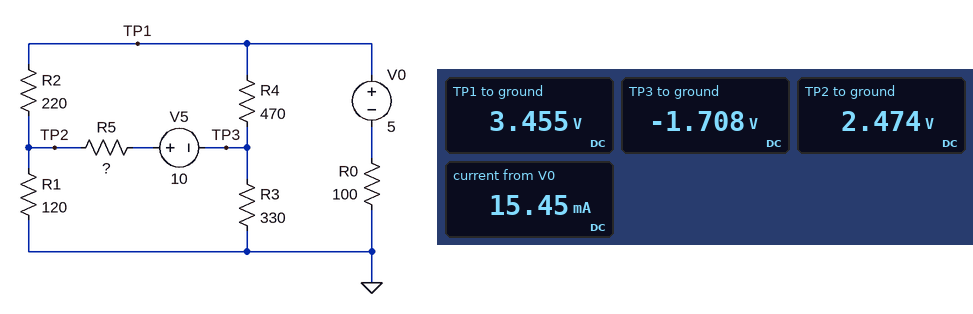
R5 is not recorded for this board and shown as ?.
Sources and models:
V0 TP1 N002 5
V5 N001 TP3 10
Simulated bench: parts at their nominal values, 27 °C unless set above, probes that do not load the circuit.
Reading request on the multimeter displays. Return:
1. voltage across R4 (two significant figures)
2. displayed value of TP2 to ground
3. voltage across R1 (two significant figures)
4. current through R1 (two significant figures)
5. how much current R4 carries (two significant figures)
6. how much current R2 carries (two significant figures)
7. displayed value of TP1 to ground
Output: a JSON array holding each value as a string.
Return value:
["5.2 V", "2.474 V", "2.5 V", "21 mA", "11 mA", "4.5 mA", "3.455 V"]
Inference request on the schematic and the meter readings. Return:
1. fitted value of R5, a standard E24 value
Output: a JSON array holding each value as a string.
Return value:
["360 Ω"]
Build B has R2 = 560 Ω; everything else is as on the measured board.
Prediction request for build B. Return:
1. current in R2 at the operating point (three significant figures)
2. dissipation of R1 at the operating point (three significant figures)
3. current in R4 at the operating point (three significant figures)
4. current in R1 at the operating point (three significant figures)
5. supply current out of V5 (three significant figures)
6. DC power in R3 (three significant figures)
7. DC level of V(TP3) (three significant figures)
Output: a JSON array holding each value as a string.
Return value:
["2.39 mA", "43.4 mW", "11.4 mA", "19.0 mA", "16.6 mA", "9.07 mW", "-1.73 V"]
